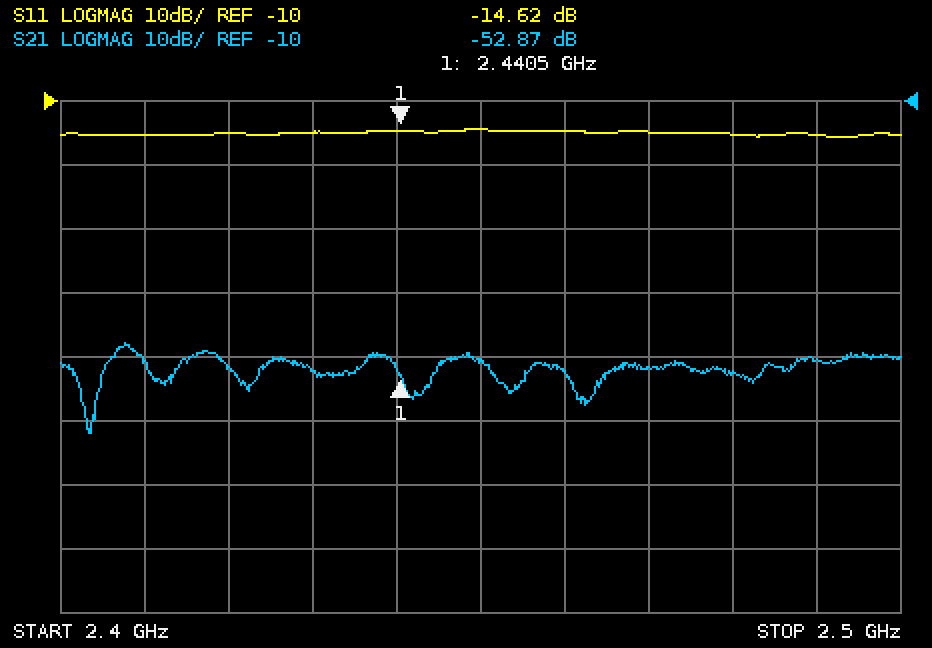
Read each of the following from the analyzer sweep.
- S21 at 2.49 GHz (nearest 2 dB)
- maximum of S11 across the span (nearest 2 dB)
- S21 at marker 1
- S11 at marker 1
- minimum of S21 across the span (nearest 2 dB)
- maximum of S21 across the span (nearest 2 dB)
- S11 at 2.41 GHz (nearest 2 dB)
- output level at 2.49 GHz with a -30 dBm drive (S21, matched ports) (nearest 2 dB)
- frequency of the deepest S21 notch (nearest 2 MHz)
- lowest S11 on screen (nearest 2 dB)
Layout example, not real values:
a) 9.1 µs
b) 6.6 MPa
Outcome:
a) -50 dB
b) -14 dB
c) -52.87 dB
d) -14.62 dB
e) -62 dB
f) -48 dB
g) -16 dB
h) -80 dBm
i) 2.404 GHz
j) -16 dB
